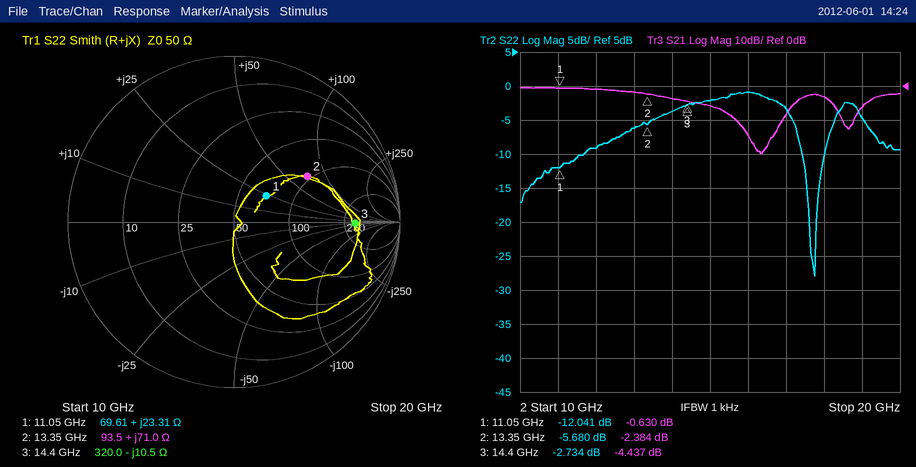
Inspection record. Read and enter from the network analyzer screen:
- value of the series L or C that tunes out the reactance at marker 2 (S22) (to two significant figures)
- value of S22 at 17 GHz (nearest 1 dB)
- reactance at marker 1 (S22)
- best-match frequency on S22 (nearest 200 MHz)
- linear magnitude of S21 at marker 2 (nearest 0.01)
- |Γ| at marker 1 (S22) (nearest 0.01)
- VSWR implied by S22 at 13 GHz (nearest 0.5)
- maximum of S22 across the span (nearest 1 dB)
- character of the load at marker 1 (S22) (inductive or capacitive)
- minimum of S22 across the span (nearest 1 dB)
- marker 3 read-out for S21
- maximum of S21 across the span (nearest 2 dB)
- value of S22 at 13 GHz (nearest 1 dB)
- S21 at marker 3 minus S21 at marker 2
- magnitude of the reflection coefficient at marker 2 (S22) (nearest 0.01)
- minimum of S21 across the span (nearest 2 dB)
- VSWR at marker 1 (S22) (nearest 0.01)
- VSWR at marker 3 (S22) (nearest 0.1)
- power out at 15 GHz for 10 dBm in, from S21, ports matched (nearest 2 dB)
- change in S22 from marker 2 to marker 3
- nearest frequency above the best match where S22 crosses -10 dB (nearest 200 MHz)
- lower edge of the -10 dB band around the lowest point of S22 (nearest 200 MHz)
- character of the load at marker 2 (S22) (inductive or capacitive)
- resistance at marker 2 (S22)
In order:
170 fF
-3 dB
+23.31 Ω
17.8 GHz
0.76
0.25
3.0
-1 dB
inductive
-28 dB
-4.437 dB
0 dB
-6 dB
-2.053 dB
0.52
-20 dB
1.67
6.4
4 dBm
2.946 dB
18.0 GHz
17.4 GHz
inductive
93.5 Ω
